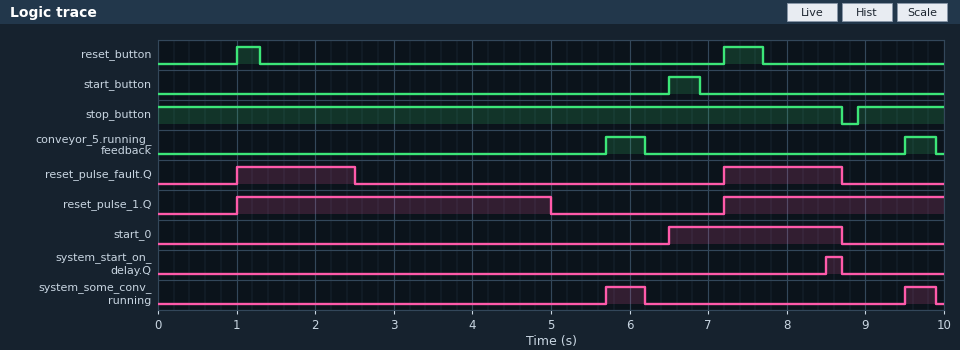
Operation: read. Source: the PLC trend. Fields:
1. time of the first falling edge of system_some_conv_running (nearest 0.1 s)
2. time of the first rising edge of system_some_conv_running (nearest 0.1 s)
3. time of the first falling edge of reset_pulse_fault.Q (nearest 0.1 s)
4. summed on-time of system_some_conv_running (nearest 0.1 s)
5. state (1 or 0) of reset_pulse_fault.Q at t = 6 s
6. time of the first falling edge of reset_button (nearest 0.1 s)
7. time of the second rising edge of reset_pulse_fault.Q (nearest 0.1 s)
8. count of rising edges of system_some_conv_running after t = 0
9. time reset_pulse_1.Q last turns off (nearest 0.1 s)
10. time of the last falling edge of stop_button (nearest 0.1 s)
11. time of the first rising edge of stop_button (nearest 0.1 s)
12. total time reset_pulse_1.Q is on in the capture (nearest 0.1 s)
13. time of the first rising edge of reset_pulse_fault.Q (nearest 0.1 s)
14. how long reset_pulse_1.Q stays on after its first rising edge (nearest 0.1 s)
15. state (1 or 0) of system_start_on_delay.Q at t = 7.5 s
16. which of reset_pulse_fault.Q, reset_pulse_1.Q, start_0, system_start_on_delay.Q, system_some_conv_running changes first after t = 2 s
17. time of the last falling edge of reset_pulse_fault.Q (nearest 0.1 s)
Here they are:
6.2 s
5.7 s
2.5 s
0.9 s
0
1.3 s
7.2 s
2
5.0 s
8.7 s
8.9 s
6.8 s
1.0 s
4.0 s
0
reset_pulse_fault.Q
8.7 s
